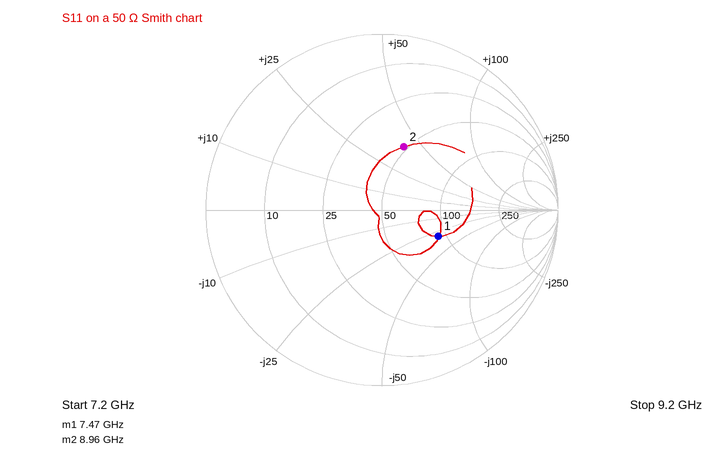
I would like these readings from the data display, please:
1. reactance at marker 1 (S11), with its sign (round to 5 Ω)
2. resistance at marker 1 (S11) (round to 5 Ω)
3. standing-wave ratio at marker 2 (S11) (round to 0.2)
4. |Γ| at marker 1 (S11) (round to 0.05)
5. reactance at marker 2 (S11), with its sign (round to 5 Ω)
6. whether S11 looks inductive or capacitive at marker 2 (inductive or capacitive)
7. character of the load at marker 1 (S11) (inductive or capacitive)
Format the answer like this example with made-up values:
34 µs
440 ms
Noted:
-30 Ω
90 Ω
2.2
0.35
+40 Ω
inductive
capacitive
